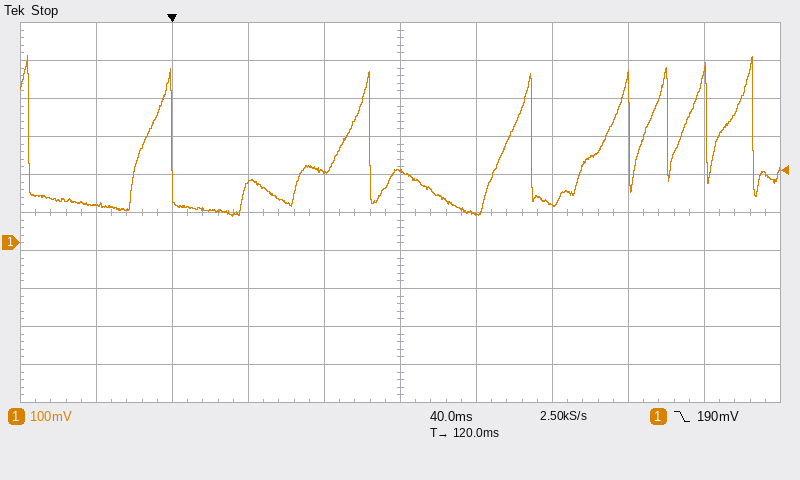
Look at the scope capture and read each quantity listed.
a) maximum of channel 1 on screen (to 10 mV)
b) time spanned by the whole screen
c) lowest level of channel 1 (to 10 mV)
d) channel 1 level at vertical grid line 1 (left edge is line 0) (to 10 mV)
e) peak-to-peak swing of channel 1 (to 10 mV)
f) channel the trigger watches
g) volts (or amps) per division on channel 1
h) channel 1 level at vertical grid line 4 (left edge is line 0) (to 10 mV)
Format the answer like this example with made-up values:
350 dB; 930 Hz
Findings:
490 mV; 400 ms; 70 mV; 100 mV; 420 mV; channel 1; 100 mV; 190 mV
